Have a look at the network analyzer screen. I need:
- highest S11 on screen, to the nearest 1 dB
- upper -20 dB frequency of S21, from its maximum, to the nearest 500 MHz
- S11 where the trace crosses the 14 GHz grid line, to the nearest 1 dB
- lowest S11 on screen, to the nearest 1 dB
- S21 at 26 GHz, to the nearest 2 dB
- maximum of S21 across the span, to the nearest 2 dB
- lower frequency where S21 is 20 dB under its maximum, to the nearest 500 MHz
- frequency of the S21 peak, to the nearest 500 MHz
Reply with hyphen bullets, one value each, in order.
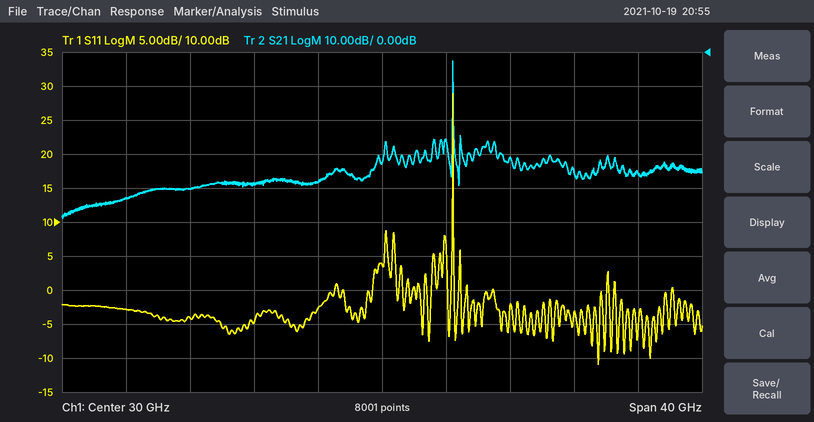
- 29 dB
- 34.5 GHz
- -3 dB
- -11 dB
- -38 dB
- -2 dB
- 34.5 GHz
- 34.5 GHz
